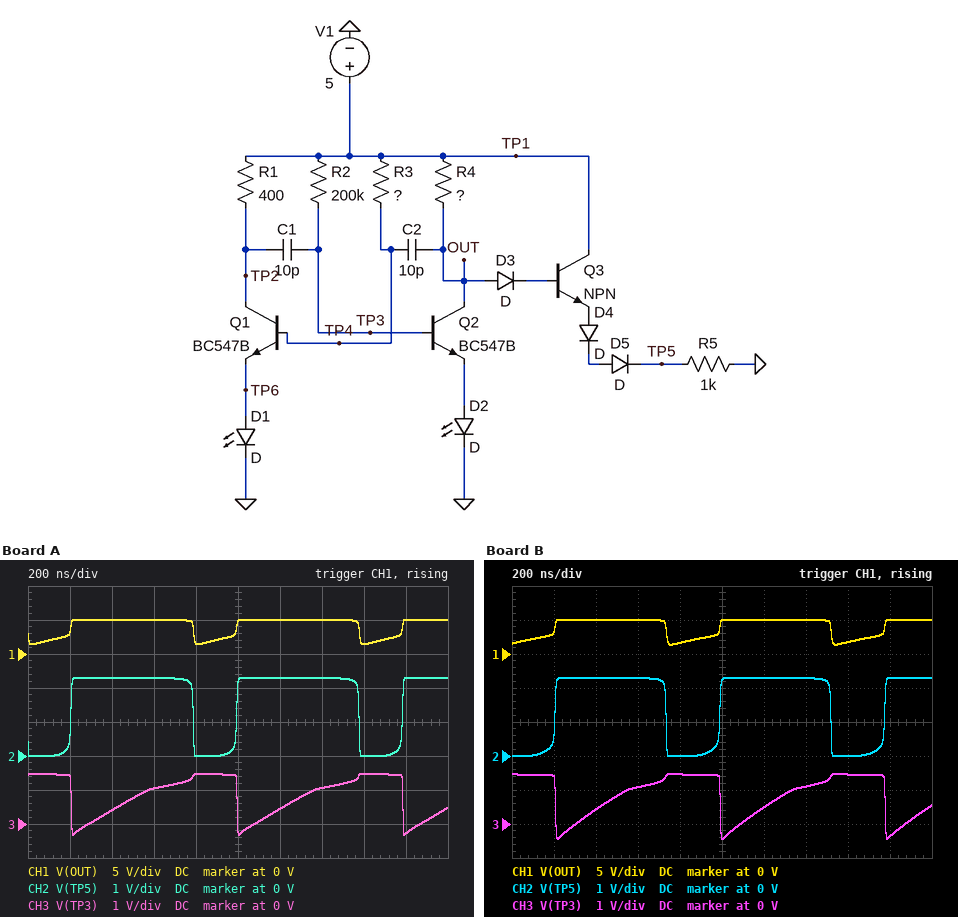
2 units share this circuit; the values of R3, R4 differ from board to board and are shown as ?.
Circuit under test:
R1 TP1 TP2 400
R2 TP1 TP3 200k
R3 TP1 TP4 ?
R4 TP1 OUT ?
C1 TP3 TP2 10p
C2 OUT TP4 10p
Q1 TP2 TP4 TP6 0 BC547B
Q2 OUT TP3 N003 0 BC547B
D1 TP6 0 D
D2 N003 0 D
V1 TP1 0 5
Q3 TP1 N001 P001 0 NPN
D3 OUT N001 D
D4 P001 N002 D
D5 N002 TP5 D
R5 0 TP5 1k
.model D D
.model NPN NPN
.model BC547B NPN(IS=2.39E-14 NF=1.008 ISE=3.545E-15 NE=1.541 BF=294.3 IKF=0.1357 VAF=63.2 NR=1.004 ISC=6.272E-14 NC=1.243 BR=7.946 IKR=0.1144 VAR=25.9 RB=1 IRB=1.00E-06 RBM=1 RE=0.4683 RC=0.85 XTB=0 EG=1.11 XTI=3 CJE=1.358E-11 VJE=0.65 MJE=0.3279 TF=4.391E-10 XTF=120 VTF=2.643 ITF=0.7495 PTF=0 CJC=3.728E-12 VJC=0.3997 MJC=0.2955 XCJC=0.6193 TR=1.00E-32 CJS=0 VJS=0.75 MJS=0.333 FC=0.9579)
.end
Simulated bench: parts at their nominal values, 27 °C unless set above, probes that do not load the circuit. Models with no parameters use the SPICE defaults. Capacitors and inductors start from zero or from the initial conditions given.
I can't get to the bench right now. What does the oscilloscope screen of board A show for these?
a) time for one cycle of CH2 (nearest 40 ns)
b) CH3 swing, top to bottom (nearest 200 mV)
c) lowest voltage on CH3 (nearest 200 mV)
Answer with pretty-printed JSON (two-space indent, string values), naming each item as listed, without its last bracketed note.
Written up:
{
  "time for one cycle of CH2": "800 ns",
  "CH3 swing, top to bottom": "1.8 V",
  "lowest voltage on CH3": "-400 mV"
}
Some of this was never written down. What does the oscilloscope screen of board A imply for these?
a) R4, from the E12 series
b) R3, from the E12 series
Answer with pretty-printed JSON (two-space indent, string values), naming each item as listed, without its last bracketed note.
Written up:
{
  "R4, from the E12 series": "150 Ω",
  "R3, from the E12 series": "150 kΩ"
}
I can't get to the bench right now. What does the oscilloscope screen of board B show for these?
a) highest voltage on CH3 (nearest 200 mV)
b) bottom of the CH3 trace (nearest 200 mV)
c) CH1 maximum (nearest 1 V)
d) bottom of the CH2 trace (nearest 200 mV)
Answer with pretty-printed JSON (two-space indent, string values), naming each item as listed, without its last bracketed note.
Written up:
{
  "highest voltage on CH3": "1.4 V",
  "bottom of the CH3 trace": "-400 mV",
  "CH1 maximum": "5 V",
  "bottom of the CH2 trace": "0 V"
}
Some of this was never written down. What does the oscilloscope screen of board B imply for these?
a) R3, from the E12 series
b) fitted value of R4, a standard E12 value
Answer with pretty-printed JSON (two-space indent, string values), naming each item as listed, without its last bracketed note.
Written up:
{
  "R3, from the E12 series": "180 kΩ",
  "fitted value of R4, a standard E12 value": "180 Ω"
}
